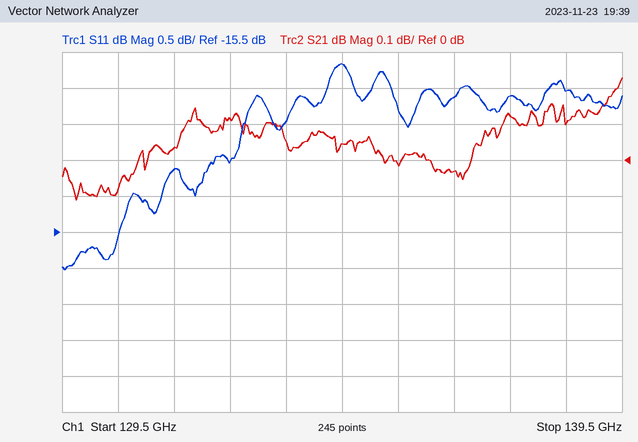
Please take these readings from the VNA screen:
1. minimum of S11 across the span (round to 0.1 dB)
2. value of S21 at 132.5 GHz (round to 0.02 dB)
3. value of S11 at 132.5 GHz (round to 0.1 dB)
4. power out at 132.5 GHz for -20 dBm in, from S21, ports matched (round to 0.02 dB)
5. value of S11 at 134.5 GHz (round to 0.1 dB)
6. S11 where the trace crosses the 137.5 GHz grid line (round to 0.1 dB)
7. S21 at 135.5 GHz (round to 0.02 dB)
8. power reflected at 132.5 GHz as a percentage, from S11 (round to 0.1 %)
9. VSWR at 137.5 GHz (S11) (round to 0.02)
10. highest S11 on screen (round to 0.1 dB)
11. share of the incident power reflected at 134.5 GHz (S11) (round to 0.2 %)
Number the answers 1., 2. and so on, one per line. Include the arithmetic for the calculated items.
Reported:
1. -16.0 dB
2. 0.12 dB
3. -14.5 dB
4. -20 dBm + (0.12 dB) = -19.88 dBm
5. -13.2 dB
6. -13.6 dB
7. -0.02 dB
8. 10^(-14.5/10) ≈ 3.5 %
9. |Γ| = 10^(-13.6/20) = 0.2089; VSWR = (1 + 0.2089)/(1 − 0.2089) ≈ 1.53, so 1.52 to the nearest 0.02
10. -13.2 dB
11. 10^(-13.2/10) ≈ 4.8 %
